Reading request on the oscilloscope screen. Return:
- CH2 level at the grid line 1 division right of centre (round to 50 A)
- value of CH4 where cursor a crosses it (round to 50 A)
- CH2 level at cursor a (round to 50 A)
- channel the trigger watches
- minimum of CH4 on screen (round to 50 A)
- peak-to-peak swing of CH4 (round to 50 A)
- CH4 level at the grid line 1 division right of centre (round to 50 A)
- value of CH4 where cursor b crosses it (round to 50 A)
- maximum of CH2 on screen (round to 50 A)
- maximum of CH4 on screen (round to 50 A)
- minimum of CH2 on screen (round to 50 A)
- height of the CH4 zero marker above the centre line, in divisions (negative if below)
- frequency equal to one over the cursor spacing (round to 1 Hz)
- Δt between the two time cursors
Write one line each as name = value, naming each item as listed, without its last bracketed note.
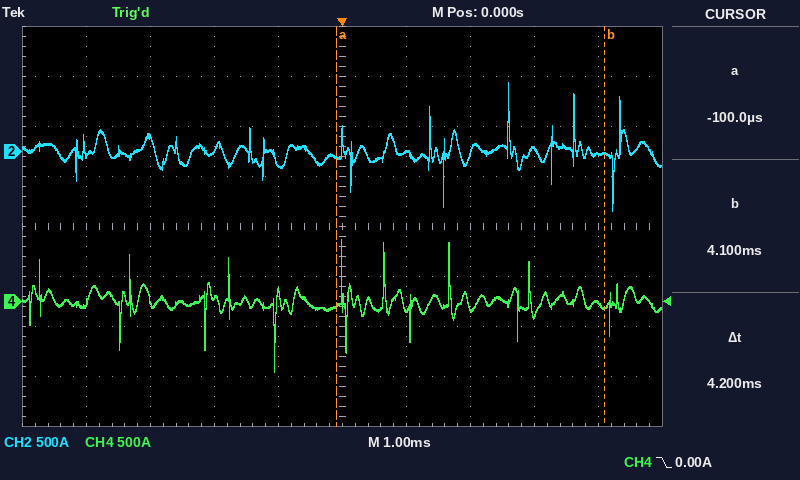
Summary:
CH2 level at the grid line 1 division right of centre = 0 A
value of CH4 where cursor a crosses it = -50 A
CH2 level at cursor a = -50 A
channel the trigger watches = CH4
minimum of CH4 on screen = -700 A
peak-to-peak swing of CH4 = 1.30 kA
CH4 level at the grid line 1 division right of centre = -50 A
value of CH4 where cursor b crosses it = -50 A
maximum of CH2 on screen = 700 A
maximum of CH4 on screen = 600 A
minimum of CH2 on screen = -600 A
height of the CH4 zero marker above the centre line, in divisions = -1.5 div
frequency equal to one over the cursor spacing = 238 Hz
Δt between the two time cursors = 4.2 ms
